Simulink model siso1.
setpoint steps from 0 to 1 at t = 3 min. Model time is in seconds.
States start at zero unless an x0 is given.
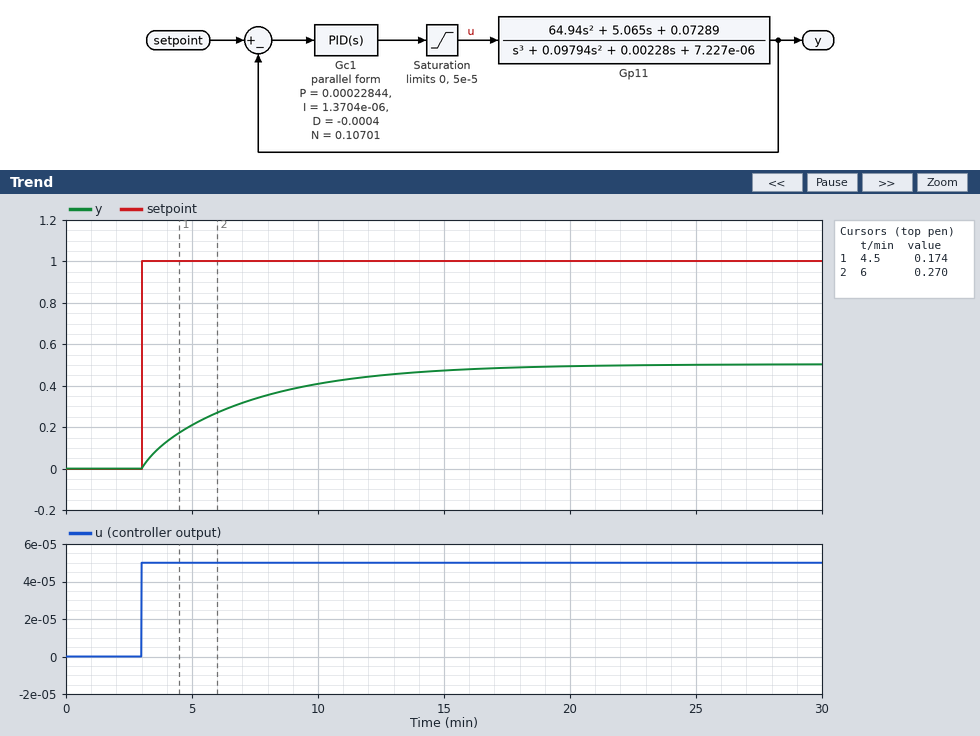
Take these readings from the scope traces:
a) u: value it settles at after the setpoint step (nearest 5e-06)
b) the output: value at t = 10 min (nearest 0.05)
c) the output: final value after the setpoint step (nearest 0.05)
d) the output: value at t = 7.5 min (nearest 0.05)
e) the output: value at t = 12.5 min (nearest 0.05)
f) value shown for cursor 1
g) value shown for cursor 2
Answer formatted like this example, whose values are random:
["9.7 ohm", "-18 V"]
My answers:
["0.000050", "0.40", "0.50", "0.35", "0.45", "0.174", "0.270"]
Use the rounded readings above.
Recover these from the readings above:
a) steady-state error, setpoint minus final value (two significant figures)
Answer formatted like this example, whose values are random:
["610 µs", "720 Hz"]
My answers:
["0.50"]
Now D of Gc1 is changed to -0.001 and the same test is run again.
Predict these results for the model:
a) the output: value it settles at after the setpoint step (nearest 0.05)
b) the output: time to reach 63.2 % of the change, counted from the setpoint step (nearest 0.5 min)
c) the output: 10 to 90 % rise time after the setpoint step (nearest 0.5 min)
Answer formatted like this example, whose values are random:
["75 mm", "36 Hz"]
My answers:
["0.50", "4.0 min", "9.5 min"]
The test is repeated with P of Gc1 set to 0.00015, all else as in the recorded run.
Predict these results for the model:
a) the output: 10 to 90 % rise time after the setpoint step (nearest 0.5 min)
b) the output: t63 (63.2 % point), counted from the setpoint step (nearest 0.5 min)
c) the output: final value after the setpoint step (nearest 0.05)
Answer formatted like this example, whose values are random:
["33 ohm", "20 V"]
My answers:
["9.5 min", "4.0 min", "0.50"]
